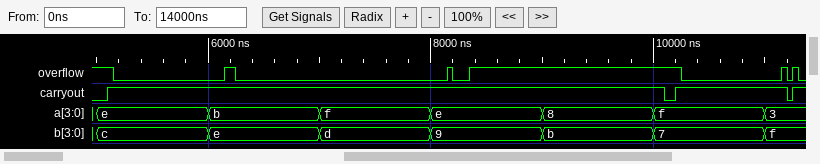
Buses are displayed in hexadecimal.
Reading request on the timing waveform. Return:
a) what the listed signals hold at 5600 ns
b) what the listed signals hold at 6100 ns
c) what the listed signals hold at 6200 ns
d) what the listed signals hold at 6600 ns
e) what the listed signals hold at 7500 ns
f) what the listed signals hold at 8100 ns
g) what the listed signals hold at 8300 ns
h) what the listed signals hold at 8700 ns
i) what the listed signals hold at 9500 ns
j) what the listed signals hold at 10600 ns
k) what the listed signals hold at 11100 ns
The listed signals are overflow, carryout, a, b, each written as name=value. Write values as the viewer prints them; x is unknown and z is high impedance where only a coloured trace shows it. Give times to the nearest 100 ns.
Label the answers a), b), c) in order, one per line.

a) overflow=0, carryout=1, a=e, b=c
b) overflow=0, carryout=1, a=b, b=e
c) overflow=1, carryout=1, a=b, b=e
d) overflow=0, carryout=1, a=b, b=e
e) overflow=0, carryout=1, a=f, b=d
f) overflow=0, carryout=1, a=e, b=9
g) overflow=0, carryout=1, a=e, b=9
h) overflow=1, carryout=1, a=e, b=9
i) overflow=1, carryout=1, a=8, b=b
j) overflow=0, carryout=1, a=f, b=7
k) overflow=0, carryout=1, a=3, b=f
